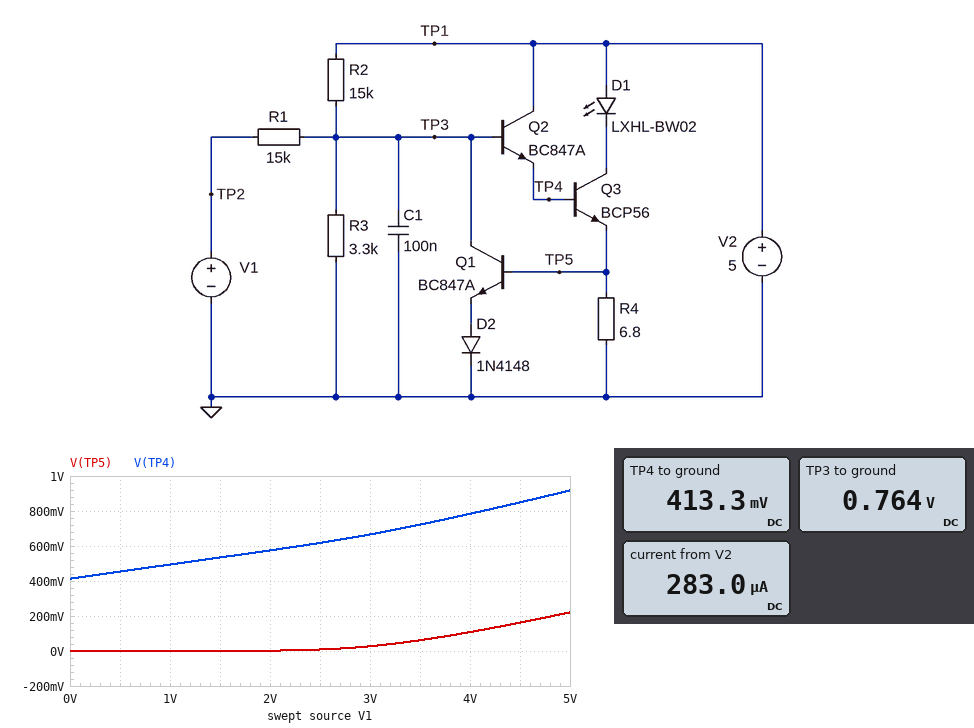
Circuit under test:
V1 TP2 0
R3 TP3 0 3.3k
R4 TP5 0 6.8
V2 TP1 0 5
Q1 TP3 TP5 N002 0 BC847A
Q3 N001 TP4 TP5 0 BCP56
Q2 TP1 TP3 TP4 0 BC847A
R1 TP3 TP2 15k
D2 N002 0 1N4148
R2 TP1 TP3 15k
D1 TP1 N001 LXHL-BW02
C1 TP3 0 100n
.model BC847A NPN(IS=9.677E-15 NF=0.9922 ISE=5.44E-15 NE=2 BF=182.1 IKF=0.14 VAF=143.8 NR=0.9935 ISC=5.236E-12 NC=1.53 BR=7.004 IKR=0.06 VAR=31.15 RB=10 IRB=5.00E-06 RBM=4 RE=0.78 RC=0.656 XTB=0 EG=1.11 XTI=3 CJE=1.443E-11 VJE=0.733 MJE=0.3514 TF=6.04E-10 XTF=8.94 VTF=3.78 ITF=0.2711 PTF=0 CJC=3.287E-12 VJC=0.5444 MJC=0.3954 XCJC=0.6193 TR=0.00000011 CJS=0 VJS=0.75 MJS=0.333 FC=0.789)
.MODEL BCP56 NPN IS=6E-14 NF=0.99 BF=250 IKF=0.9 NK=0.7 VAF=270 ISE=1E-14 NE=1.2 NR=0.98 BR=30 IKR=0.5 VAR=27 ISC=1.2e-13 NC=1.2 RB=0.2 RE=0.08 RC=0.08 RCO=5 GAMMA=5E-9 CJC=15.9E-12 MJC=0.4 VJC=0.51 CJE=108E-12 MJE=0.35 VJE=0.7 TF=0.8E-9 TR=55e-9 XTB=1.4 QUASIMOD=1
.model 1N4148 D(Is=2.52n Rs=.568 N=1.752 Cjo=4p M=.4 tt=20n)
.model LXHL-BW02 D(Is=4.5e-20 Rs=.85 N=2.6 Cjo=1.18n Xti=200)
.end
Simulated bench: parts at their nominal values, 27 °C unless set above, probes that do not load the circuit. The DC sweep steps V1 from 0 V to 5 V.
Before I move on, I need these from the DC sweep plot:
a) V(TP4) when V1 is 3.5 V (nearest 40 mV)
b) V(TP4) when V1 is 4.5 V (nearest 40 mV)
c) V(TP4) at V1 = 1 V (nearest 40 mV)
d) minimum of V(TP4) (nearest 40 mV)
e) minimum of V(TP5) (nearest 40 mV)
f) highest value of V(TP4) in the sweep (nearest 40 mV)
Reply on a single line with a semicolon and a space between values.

720 mV; 840 mV; 480 mV; 400 mV; 0 V; 920 mV
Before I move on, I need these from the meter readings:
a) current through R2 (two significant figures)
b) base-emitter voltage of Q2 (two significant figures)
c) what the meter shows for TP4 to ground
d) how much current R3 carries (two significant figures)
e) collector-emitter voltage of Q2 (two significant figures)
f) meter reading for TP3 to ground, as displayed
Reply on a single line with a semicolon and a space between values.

280 µA; 350 mV; 413.3 mV; 230 µA; 4.6 V; 0.764 V
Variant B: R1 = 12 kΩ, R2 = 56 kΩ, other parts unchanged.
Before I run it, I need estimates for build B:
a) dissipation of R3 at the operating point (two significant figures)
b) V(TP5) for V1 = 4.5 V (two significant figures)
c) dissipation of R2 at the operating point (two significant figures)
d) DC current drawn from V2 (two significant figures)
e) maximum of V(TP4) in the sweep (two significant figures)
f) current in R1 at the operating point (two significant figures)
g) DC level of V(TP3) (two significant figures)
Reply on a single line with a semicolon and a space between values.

15 µW; 9.0 mV; 410 µW; 85 µA; 690 mV; 18 µA; 220 mV
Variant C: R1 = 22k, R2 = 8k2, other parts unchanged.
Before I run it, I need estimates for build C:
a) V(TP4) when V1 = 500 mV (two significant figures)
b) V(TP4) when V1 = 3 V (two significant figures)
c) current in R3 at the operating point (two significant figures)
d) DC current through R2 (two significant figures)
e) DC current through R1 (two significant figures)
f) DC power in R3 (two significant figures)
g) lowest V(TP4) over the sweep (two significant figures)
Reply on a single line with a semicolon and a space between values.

760 mV; 970 mV; 390 µA; 450 µA; 59 µA; 510 µW; 720 mV
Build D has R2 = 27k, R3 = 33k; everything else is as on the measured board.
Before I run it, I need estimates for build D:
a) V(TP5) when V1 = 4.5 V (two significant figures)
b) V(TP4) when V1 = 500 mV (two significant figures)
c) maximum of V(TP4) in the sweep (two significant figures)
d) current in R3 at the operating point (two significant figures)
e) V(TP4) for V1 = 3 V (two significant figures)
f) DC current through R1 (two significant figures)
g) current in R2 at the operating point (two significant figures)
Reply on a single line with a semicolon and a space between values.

1.1 V; 1.0 V; 1.9 V; 42 µA; 1.8 V; 92 µA; 130 µA
